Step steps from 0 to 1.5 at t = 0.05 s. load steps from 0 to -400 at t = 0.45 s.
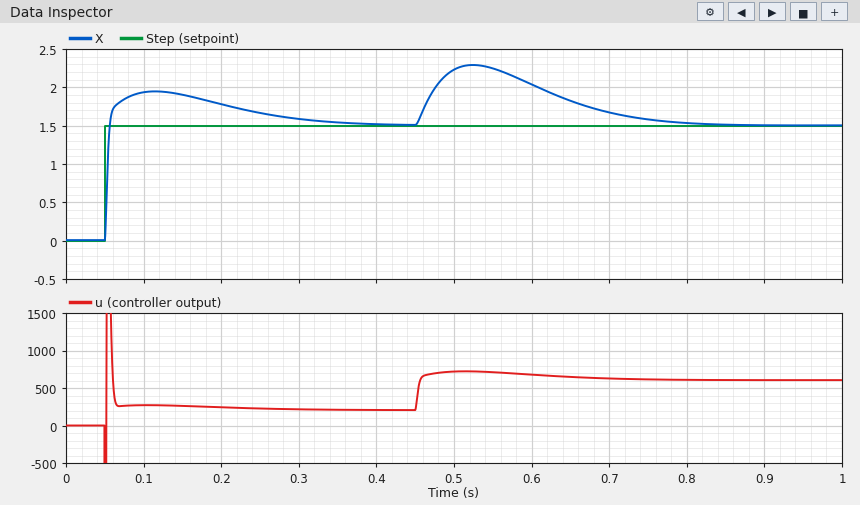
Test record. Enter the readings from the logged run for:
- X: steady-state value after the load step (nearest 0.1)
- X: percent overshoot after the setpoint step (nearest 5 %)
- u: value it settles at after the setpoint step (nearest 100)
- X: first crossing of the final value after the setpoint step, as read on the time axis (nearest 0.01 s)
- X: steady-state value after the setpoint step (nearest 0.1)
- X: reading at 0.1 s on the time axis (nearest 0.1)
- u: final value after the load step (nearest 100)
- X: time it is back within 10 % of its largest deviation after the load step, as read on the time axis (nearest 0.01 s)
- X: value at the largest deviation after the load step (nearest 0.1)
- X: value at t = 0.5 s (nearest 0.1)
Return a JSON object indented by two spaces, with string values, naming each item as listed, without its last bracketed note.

{
  "X: steady-state value after the load step": "1.5",
  "X: percent overshoot after the setpoint step": "30 %",
  "u: value it settles at after the setpoint step": "200",
  "X: first crossing of the final value after the setpoint step, as read on the time axis": "0.06 s",
  "X: steady-state value after the setpoint step": "1.5",
  "X: reading at 0.1 s on the time axis": "1.9",
  "u: final value after the load step": "600",
  "X: time it is back within 10 % of its largest deviation after the load step, as read on the time axis": "0.75 s",
  "X: value at the largest deviation after the load step": "2.3",
  "X: value at t = 0.5 s": "2.2"
}
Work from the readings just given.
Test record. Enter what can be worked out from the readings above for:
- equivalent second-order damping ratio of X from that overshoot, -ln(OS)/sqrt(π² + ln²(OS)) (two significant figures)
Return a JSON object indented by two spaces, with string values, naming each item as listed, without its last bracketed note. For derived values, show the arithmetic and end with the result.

{
  "equivalent second-order damping ratio of X from that overshoot, -ln(OS)/sqrt(π² + ln²(OS))": "ln(0.3) = -1.204; 1.204 / sqrt(9.870 + 1.450) = 0.36"
}
